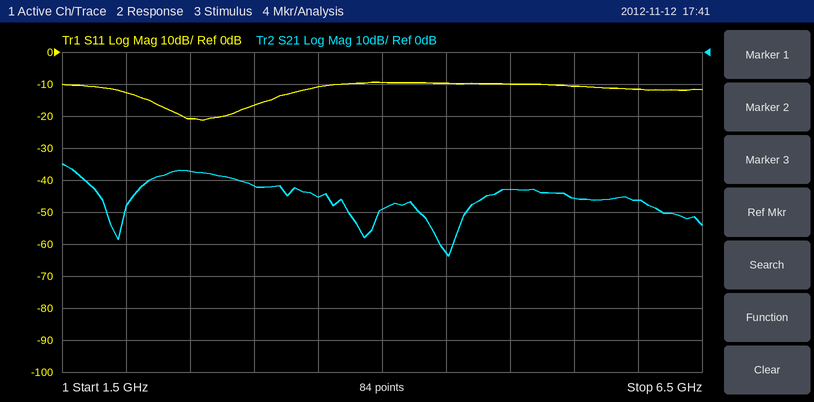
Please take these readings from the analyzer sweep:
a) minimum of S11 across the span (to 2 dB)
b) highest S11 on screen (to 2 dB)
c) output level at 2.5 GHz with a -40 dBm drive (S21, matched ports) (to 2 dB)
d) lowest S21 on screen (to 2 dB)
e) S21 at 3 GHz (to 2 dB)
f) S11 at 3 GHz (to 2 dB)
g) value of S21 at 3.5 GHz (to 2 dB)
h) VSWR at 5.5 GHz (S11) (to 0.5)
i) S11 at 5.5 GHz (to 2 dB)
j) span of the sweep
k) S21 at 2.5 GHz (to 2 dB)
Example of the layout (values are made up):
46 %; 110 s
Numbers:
-22 dB; -10 dB; -78 dBm; -64 dB; -42 dB; -16 dB; -46 dB; 2.0; -10 dB; 5 GHz; -38 dB
